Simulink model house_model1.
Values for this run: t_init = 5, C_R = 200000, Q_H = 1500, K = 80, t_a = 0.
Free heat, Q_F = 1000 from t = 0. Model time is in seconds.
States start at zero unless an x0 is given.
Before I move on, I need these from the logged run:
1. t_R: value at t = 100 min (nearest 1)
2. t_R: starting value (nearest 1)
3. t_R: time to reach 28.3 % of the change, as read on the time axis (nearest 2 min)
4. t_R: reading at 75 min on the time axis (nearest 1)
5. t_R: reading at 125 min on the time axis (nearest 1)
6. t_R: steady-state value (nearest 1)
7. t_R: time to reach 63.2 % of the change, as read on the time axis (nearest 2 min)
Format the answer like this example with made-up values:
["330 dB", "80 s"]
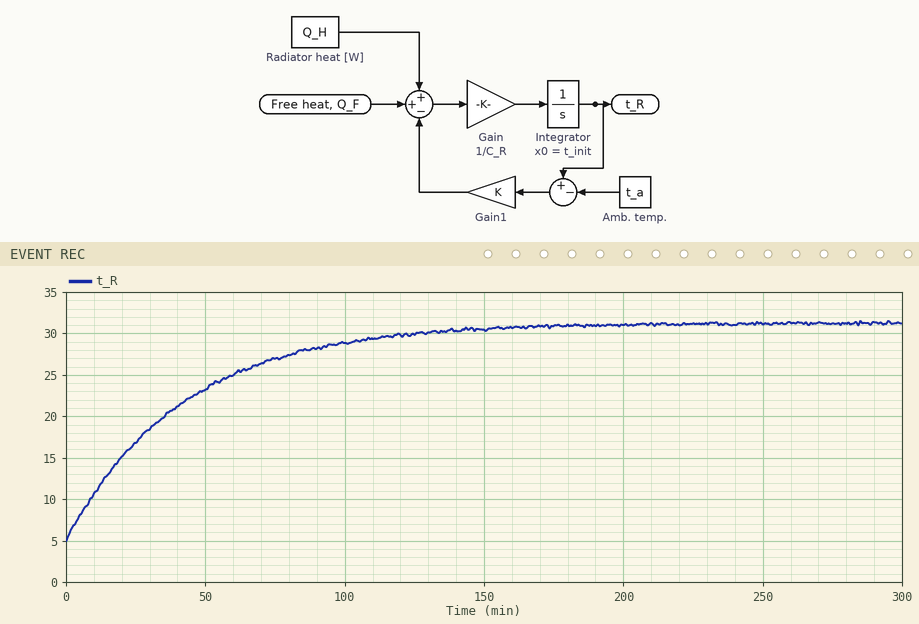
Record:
["29", "5", "14 min", "27", "30", "31", "42 min"]
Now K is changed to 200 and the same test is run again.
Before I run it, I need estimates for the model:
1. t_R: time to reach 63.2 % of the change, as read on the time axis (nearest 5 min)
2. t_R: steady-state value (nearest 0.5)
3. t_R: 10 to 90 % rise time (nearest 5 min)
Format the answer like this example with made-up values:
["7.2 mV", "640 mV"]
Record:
["15 min", "12.5", "35 min"]
